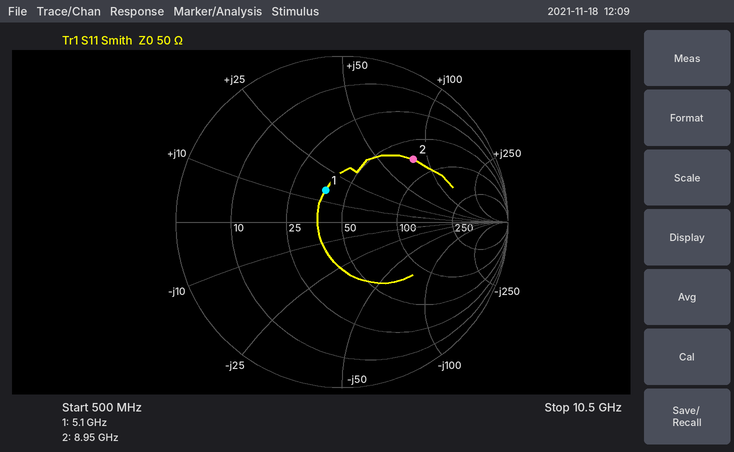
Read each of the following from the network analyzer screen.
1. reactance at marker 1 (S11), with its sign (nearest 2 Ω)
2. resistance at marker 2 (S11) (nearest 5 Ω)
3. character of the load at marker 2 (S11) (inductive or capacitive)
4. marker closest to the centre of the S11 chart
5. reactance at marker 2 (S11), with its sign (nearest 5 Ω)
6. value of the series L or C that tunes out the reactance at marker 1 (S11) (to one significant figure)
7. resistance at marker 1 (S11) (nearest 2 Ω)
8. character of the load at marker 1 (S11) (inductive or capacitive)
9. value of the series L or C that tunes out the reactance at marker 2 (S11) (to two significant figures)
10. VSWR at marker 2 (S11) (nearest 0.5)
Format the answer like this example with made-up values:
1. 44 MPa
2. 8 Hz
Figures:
1. +16 Ω
2. 70 Ω
3. inductive
4. marker 1
5. +80 Ω
6. 2 pF
7. 38 Ω
8. inductive
9. 220 fF
10. 3.5
